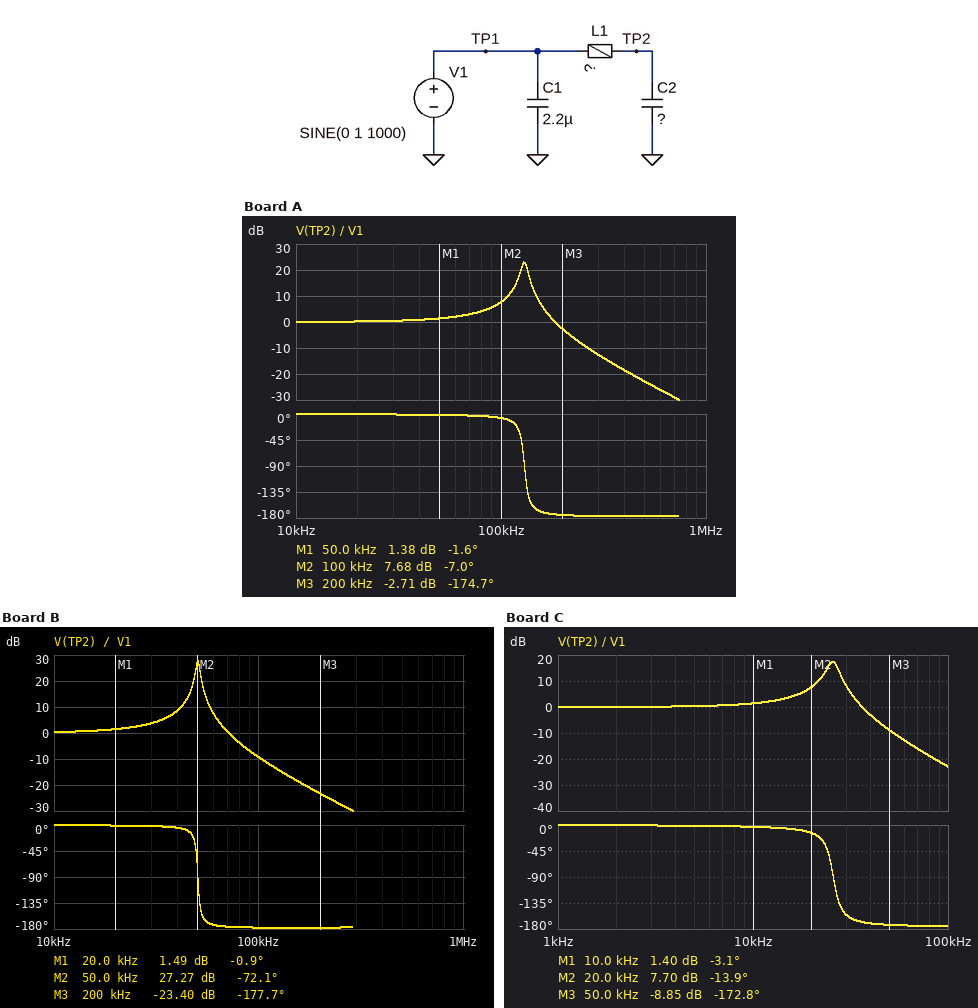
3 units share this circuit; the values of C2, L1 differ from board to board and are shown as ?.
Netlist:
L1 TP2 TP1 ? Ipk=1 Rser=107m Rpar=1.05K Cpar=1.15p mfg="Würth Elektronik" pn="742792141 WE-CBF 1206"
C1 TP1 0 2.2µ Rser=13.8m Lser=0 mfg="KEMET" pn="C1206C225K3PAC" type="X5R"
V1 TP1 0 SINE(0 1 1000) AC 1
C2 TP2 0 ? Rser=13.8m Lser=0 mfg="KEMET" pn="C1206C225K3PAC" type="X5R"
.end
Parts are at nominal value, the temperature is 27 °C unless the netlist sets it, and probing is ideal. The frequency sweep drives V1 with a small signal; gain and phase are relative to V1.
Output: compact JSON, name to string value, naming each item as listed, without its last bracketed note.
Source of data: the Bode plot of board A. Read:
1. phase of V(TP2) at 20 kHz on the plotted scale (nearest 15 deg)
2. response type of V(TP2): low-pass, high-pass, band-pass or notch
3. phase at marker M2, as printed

{"phase of V(TP2) at 20 kHz on the plotted scale": "0 deg", "response type of V(TP2): low-pass, high-pass, band-pass or notch": "low-pass", "phase at marker M2, as printed": "-7.0 deg"}
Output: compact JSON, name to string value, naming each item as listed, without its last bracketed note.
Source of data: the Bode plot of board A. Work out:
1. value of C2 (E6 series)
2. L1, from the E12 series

{"value of C2": "680 nF", "L1, from the E12 series": "2.2 µH"}
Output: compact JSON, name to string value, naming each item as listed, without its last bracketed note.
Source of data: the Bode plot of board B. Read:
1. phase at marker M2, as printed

{"phase at marker M2, as printed": "-72.1 deg"}
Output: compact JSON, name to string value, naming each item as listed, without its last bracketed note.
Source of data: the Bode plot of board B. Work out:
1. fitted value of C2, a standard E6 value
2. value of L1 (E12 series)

{"fitted value of C2, a standard E6 value": "1 µF", "value of L1": "10 µH"}
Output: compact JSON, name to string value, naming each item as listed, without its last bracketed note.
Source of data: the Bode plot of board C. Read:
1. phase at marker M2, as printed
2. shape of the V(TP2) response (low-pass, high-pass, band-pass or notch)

{"phase at marker M2, as printed": "-13.9 deg", "shape of the V(TP2) response": "low-pass"}
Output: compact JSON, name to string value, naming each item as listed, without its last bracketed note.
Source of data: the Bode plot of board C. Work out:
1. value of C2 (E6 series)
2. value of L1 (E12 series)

{"value of C2": "6.8 µF", "value of L1": "5.6 µH"}
